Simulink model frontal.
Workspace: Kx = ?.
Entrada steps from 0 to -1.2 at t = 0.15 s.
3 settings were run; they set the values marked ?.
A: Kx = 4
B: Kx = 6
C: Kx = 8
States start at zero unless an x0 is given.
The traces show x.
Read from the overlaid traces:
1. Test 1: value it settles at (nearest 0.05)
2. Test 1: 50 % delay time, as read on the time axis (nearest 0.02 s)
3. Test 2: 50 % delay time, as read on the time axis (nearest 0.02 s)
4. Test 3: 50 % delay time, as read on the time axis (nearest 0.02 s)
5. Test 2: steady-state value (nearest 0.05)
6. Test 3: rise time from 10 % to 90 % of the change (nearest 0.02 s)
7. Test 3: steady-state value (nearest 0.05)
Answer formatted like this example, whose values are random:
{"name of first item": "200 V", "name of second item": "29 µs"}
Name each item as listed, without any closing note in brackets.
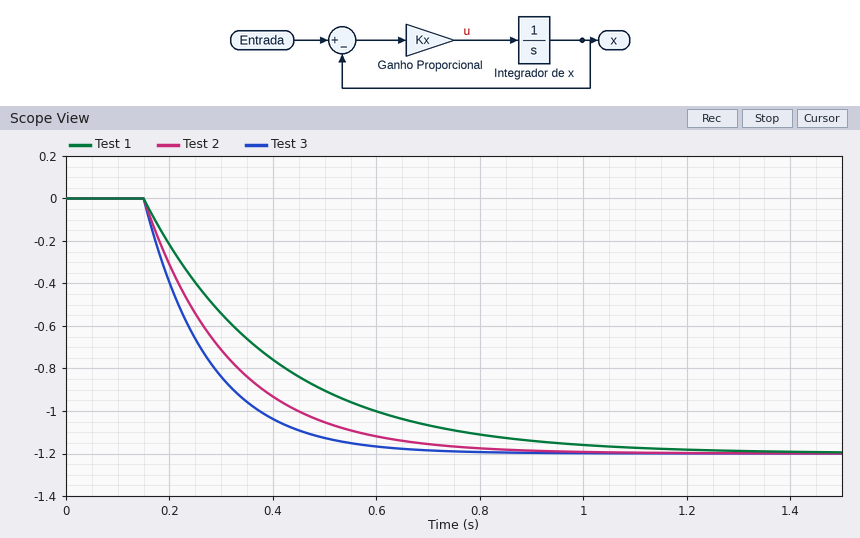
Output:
{"Test 1: value it settles at": "-1.20", "Test 1: 50 % delay time, as read on the time axis": "0.32 s", "Test 2: 50 % delay time, as read on the time axis": "0.26 s", "Test 3: 50 % delay time, as read on the time axis": "0.24 s", "Test 2: steady-state value": "-1.20", "Test 3: rise time from 10 % to 90 % of the change": "0.28 s", "Test 3: steady-state value": "-1.20"}
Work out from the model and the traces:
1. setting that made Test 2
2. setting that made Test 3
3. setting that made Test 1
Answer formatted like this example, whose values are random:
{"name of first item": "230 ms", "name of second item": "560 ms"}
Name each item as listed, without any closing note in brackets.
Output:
{"setting that made Test 2": "B", "setting that made Test 3": "C", "setting that made Test 1": "A"}
